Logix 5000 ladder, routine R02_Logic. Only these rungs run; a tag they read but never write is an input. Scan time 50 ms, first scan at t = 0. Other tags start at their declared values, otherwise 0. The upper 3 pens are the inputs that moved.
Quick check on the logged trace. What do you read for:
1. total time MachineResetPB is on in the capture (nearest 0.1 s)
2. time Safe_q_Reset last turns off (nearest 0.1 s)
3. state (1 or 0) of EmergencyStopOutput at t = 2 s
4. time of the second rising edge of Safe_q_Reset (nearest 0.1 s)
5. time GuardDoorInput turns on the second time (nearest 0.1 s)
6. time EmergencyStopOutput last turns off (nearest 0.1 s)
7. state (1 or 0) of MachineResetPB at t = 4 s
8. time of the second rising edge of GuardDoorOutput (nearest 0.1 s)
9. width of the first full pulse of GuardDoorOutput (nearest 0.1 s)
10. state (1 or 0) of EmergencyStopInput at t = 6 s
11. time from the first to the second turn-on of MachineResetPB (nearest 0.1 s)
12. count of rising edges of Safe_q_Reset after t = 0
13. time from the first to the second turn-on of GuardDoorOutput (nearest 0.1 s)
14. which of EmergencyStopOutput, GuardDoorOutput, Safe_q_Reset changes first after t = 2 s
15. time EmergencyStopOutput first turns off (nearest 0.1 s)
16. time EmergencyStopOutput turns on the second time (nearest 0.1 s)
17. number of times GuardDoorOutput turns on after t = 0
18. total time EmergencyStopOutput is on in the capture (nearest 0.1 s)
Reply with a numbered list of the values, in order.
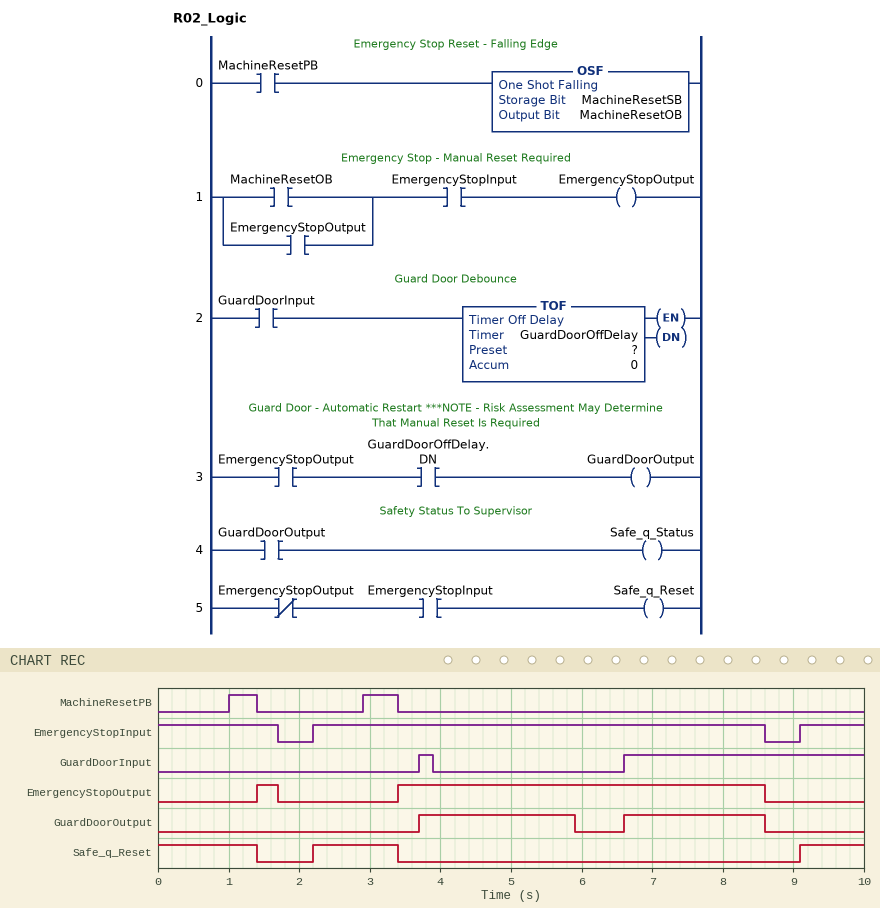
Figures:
1. 0.9 s
2. 3.4 s
3. 0
4. 9.1 s
5. 6.6 s
6. 8.6 s
7. 0
8. 6.6 s
9. 2.2 s
10. 1
11. 1.9 s
12. 2
13. 2.9 s
14. Safe_q_Reset
15. 1.7 s
16. 3.4 s
17. 2
18. 5.5 s
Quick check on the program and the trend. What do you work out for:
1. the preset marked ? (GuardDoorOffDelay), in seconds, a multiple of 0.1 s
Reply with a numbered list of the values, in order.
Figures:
1. 2.0 s
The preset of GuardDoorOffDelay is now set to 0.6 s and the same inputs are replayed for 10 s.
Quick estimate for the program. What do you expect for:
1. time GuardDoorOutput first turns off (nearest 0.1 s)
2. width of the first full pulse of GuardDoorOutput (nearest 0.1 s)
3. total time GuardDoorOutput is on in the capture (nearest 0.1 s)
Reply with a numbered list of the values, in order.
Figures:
1. 4.5 s
2. 0.8 s
3. 2.8 s
